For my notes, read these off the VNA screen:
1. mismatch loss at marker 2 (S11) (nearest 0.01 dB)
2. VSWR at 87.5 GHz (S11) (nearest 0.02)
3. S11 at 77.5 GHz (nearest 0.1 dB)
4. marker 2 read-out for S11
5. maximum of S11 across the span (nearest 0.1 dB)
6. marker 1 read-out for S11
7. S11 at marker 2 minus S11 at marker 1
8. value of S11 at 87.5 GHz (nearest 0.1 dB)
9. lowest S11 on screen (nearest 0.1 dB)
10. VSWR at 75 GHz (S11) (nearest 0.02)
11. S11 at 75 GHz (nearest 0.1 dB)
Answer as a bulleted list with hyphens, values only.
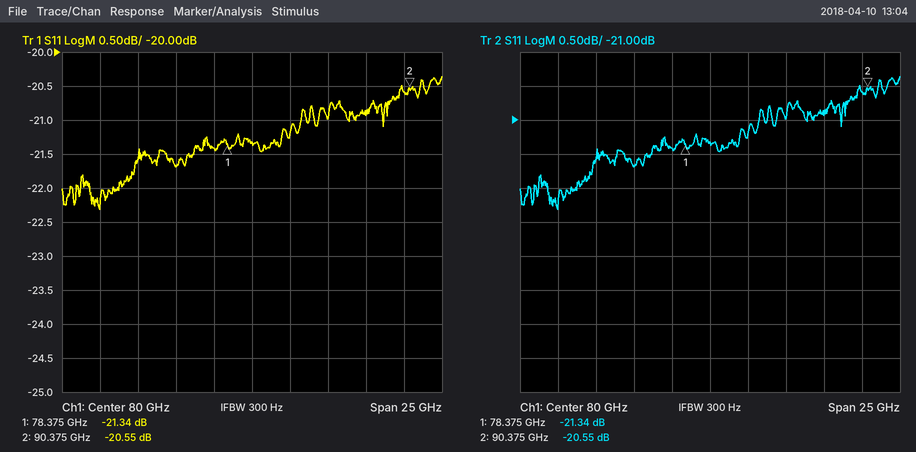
- 0.04 dB
- 1.20
- -21.4 dB
- -20.55 dB
- -20.4 dB
- -21.34 dB
- 0.79 dB
- -20.9 dB
- -22.3 dB
- 1.18
- -21.7 dB
